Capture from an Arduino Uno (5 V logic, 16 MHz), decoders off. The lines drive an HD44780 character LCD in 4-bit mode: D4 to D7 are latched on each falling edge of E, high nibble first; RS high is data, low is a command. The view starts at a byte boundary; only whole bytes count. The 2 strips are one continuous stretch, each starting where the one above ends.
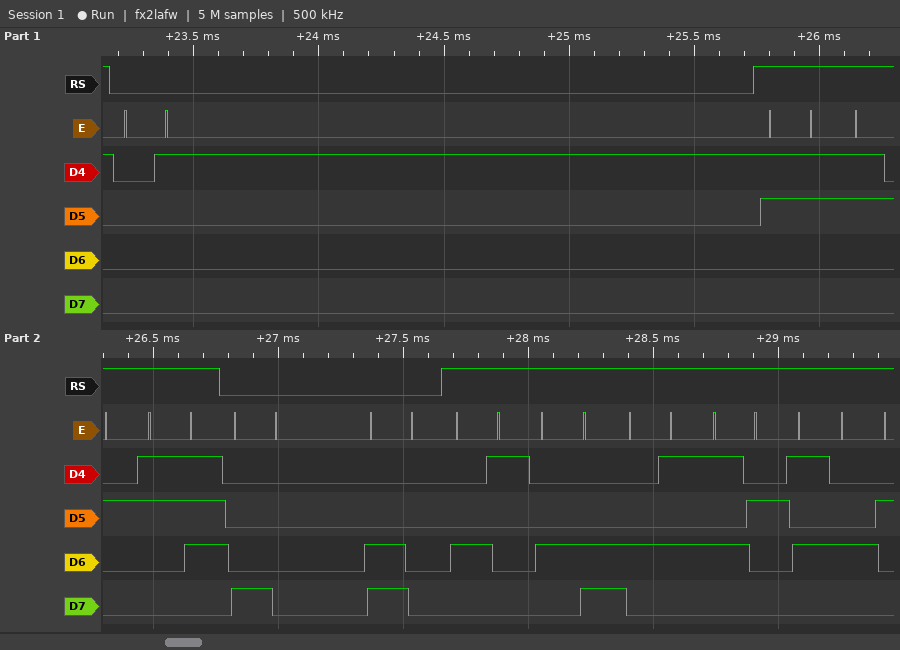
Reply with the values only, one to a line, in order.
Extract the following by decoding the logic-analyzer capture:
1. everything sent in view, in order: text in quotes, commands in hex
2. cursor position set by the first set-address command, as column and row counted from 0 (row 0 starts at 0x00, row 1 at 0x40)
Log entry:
0x01 "327" 0x80 0xC0 "ALERT"
column 0, row 0
